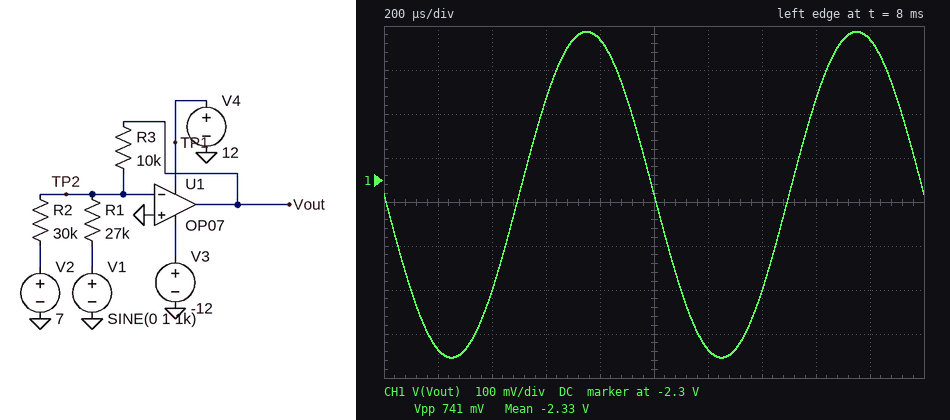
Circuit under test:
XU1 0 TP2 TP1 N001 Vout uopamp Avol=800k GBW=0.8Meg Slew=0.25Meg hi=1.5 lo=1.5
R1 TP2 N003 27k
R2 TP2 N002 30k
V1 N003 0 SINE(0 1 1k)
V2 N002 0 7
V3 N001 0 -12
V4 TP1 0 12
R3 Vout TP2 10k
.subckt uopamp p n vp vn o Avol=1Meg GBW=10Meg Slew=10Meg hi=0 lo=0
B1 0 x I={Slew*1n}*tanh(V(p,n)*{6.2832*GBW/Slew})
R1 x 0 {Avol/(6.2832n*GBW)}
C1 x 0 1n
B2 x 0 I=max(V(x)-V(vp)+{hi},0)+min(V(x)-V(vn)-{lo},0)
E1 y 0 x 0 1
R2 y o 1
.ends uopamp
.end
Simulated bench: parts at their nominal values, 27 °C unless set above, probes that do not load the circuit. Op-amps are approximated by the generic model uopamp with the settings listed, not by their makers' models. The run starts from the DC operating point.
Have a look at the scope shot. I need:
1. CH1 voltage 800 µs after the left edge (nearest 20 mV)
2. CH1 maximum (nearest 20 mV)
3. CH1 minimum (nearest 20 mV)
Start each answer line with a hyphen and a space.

- -1.98 V
- -1.96 V
- -2.70 V
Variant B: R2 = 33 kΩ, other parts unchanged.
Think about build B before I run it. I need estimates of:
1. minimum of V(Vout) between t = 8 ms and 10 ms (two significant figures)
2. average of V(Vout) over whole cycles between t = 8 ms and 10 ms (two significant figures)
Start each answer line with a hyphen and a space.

- -2.5 V
- -2.1 V
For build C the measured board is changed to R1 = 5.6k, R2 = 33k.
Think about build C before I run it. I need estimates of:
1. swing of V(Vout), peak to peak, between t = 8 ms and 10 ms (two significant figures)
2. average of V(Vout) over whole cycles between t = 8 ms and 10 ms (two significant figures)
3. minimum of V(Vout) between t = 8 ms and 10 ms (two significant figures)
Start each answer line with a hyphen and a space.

- 3.6 V
- -2.1 V
- -3.9 V
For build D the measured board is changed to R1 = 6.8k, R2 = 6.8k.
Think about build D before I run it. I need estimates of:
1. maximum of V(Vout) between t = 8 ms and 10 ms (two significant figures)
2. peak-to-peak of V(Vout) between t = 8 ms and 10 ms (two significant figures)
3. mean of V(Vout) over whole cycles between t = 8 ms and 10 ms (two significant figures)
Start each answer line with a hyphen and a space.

- -8.8 V
- 1.7 V
- -9.9 V
